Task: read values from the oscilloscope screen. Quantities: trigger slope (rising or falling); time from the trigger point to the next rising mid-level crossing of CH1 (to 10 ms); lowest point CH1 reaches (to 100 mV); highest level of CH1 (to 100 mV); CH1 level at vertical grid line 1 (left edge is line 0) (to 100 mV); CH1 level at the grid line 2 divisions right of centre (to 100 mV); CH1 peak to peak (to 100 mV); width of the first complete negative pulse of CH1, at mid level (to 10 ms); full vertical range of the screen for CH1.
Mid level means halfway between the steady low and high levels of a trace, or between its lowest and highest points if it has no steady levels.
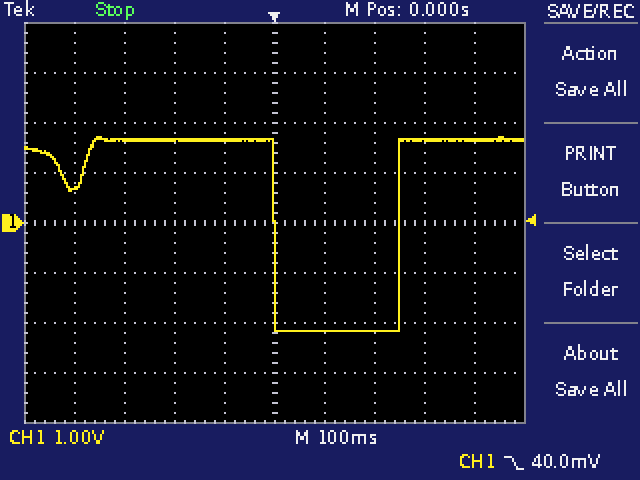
falling
250 ms
-2.2 V
1.7 V
700 mV
-2.2 V
3.9 V
250 ms
8 V
